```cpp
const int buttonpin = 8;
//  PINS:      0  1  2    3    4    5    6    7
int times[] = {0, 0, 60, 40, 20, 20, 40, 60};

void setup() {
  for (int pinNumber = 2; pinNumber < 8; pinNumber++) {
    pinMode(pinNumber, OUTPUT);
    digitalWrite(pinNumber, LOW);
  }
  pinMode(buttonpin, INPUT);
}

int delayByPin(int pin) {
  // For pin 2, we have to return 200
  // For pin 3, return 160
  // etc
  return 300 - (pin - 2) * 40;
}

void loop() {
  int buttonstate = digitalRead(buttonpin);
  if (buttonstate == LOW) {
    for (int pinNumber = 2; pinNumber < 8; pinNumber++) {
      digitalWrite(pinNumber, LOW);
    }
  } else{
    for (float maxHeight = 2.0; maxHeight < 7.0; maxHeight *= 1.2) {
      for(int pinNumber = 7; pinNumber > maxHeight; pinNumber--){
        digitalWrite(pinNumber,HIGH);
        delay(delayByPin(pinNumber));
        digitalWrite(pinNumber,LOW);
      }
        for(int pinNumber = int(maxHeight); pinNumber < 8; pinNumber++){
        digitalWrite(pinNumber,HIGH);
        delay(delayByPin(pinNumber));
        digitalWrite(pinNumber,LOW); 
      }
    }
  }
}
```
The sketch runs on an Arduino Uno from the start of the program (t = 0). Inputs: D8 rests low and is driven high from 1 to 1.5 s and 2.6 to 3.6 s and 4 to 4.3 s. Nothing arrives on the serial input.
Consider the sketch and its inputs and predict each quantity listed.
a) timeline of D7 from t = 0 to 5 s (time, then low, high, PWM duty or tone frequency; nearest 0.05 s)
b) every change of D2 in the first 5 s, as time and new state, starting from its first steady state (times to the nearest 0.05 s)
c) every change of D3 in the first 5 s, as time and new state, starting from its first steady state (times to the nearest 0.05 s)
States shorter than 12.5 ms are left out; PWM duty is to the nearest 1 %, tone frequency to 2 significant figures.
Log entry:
0 s low; 1 s high; 1.1 s low; 3 s high; 3.2 s low
0 s low; 1.9 s high; 2.2 s low; 4 s high; 4.3 s low
0 s low; 1.65 s high; 1.9 s low; 2.2 s high; 2.45 s low; 3.75 s high; 4 s low; 4.3 s high; 4.55 s low
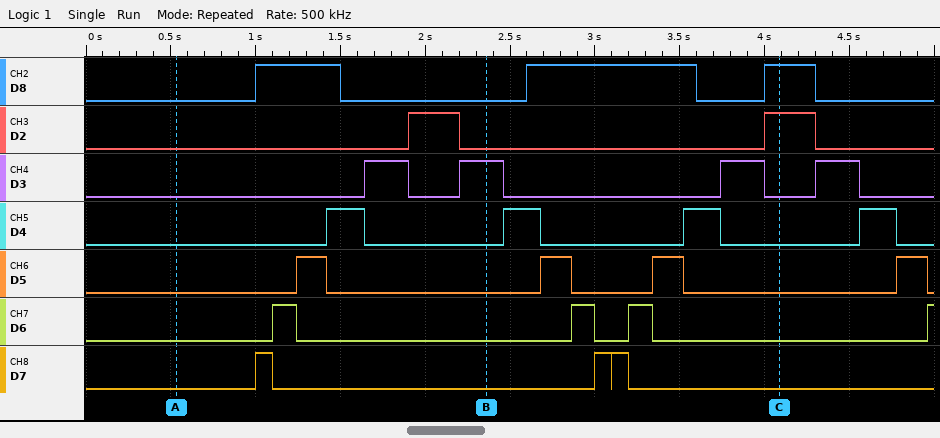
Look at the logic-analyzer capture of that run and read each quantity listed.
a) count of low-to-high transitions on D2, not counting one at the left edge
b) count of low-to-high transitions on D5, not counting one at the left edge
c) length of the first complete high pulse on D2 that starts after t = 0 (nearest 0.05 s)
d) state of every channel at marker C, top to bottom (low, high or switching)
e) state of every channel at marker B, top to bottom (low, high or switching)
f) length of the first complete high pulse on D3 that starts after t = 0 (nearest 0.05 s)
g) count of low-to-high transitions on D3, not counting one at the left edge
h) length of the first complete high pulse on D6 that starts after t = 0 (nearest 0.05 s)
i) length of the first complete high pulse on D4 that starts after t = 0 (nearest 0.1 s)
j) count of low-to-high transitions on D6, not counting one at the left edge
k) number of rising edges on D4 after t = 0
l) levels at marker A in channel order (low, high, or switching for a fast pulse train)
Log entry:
2
4
0.30 s
D8 high, D2 high, D3 low, D4 low, D5 low, D6 low, D7 low
D8 low, D2 low, D3 high, D4 low, D5 low, D6 low, D7 low
0.25 s
4
0.15 s
0.2 s
4
4
D8 low, D2 low, D3 low, D4 low, D5 low, D6 low, D7 low
